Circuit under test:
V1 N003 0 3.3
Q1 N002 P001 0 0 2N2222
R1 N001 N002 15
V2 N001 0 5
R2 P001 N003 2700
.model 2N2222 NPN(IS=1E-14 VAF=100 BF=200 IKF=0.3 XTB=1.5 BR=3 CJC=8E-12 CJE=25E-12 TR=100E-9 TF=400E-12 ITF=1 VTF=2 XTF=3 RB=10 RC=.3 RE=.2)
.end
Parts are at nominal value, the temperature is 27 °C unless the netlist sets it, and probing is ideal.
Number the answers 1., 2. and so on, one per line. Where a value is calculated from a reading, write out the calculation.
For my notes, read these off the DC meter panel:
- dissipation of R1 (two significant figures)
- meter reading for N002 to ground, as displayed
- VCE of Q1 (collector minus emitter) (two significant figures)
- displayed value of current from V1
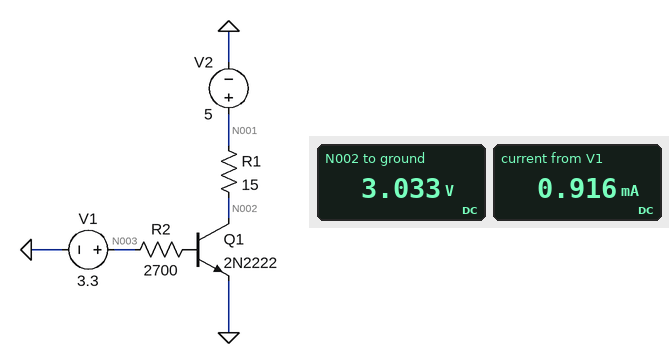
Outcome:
1. (5 V - 3.033 V)^2 / 15 Ω = 260 mW
2. 3.033 V
3. 3.033 V = 3.0 V
4. 0.916 mA
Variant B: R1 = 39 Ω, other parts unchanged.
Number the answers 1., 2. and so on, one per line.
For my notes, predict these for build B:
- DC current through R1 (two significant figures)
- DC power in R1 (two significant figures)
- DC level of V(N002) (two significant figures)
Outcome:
1. 120 mA
2. 580 mW
3. 240 mV
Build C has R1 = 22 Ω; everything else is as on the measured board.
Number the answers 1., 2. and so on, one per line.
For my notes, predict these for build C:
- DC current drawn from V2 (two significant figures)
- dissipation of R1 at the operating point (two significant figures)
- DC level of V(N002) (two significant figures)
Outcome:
1. 130 mA
2. 370 mW
3. 2.1 V
